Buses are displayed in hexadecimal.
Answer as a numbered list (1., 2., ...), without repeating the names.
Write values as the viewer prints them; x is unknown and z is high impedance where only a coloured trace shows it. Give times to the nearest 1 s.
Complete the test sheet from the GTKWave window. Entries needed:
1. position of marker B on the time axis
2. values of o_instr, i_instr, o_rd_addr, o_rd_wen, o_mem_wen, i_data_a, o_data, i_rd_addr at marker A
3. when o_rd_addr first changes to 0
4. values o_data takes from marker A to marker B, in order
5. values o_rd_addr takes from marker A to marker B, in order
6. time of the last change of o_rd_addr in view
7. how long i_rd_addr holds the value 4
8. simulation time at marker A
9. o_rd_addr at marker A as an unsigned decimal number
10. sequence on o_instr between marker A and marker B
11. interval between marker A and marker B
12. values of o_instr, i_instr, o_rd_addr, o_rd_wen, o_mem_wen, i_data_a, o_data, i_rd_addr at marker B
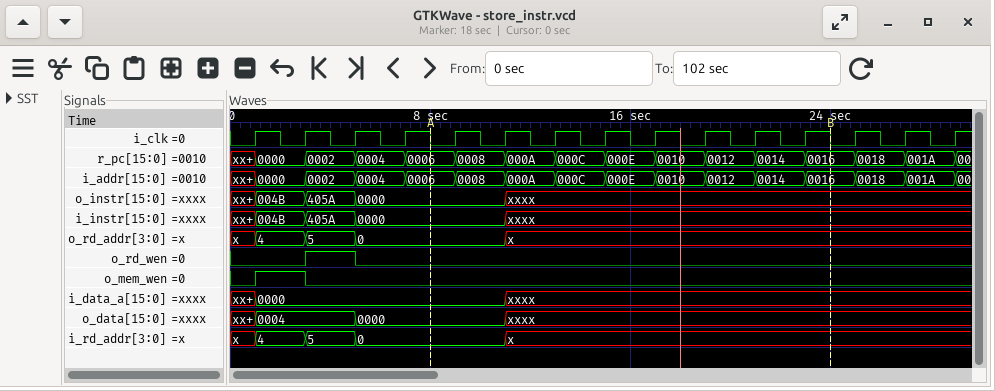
1. 24 s
2. o_instr=0000, i_instr=0000, o_rd_addr=0, o_rd_wen=0, o_mem_wen=0, i_data_a=0000, o_data=0000, i_rd_addr=0
3. 5 s
4. 0000, xxxx
5. 0, x
6. 11 s
7. 2 s
8. 8 s
9. 0
10. 0000, xxxx
11. 16 s
12. o_instr=xxxx, i_instr=xxxx, o_rd_addr=x, o_rd_wen=0, o_mem_wen=0, i_data_a=xxxx, o_data=xxxx, i_rd_addr=x
